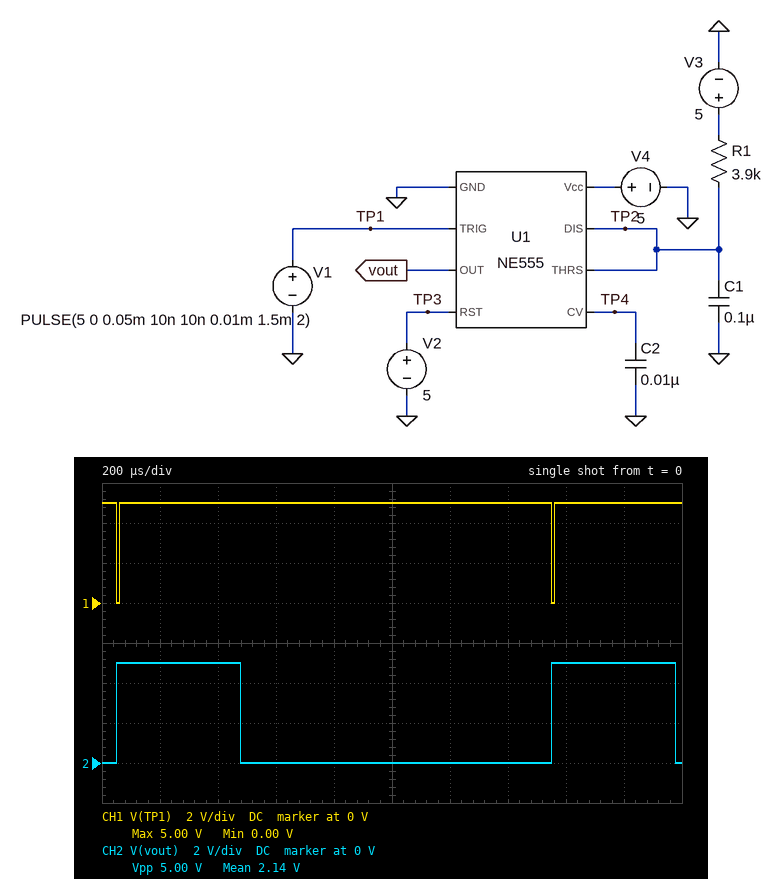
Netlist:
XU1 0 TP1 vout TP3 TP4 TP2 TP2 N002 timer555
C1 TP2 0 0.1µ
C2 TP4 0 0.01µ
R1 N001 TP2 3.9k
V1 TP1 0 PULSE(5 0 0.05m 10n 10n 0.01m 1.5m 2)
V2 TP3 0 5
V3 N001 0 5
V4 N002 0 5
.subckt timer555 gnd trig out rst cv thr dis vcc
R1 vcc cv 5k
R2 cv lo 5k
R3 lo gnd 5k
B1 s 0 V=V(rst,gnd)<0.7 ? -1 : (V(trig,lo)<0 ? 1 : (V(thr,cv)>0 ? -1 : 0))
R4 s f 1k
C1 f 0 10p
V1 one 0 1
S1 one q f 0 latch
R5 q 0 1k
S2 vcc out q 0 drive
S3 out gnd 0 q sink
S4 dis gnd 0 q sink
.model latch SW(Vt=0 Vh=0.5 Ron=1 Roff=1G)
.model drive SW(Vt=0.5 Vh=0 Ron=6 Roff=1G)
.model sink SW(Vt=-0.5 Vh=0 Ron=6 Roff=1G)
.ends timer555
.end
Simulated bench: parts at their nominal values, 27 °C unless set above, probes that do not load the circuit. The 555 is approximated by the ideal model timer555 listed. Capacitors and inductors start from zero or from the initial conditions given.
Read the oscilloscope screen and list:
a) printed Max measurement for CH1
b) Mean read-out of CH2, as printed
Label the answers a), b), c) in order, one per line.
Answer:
a) 5.00 V
b) 2.14 V
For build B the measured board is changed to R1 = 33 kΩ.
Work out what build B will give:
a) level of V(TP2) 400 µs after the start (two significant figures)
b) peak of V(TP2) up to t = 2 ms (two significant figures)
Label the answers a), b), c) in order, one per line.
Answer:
a) 500 mV
b) 2.2 V
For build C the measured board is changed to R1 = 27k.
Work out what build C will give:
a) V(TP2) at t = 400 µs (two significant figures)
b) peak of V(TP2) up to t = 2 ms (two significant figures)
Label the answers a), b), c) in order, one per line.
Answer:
a) 610 mV
b) 2.6 V
